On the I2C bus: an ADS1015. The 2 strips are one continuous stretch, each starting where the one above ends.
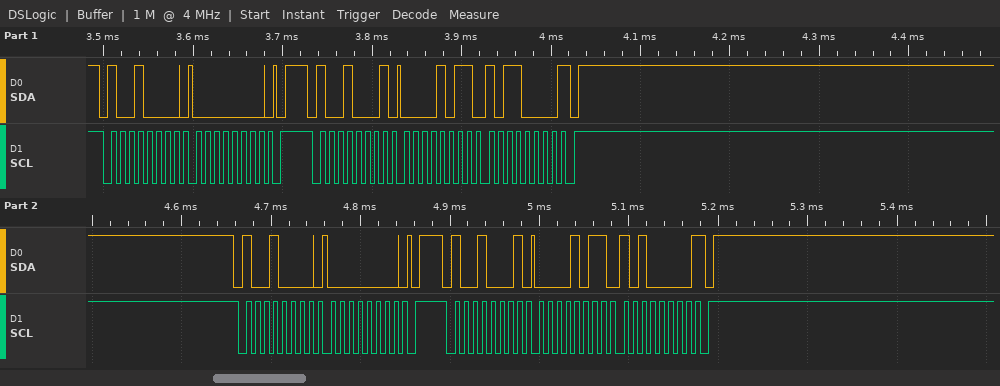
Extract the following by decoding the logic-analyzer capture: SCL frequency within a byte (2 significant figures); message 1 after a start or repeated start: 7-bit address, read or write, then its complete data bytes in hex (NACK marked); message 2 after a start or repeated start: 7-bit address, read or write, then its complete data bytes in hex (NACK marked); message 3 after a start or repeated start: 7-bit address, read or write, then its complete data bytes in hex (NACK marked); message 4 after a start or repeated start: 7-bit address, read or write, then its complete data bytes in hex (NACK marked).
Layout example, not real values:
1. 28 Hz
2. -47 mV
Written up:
1. 100 kHz
2. 0x48 write: 00
3. 0x48 read: 0B B0 NACK
4. 0x48 write: 00
5. 0x48 read: 0B A0 NACK
